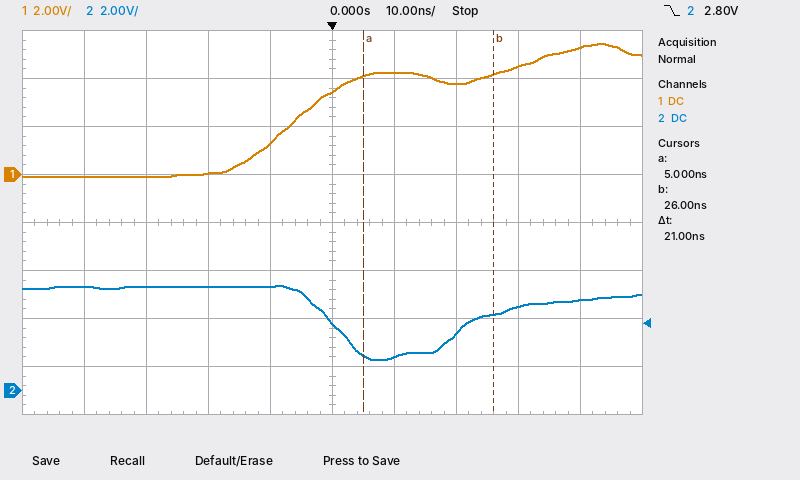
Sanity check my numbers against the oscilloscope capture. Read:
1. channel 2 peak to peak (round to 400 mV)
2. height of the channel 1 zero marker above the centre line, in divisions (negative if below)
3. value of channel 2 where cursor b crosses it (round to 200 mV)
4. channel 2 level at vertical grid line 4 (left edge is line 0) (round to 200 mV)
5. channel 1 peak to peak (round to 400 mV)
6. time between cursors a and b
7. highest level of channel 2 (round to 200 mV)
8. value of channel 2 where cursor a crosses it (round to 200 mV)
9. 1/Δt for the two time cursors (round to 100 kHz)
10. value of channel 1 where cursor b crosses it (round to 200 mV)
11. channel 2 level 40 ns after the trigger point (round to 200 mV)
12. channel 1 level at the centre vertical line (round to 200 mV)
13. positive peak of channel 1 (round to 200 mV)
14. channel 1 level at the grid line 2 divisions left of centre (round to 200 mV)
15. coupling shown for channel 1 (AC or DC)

3.2 V
+1.0 div
3.2 V
4.4 V
5.6 V
21 ns
4.4 V
1.4 V
47.6 MHz
4.2 V
3.8 V
3.4 V
5.4 V
0.0 V
DC
